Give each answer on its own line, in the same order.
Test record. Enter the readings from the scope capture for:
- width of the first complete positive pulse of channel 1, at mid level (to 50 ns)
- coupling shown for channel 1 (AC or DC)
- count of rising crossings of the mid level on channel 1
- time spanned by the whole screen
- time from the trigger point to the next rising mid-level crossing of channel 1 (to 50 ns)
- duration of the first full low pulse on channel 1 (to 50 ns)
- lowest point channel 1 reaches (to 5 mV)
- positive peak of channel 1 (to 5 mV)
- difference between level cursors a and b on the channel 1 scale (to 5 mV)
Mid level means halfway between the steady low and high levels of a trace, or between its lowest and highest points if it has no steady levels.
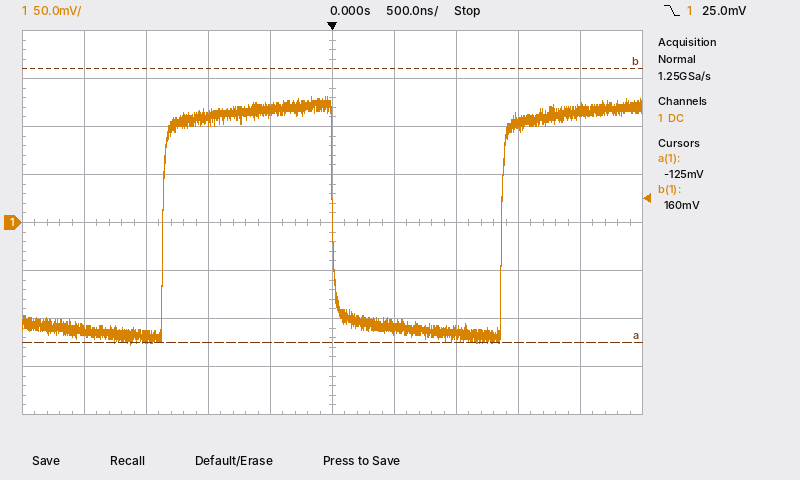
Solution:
1.35 µs
DC
2
5 µs
1.35 µs
1.35 µs
-125 mV
130 mV
285 mV
